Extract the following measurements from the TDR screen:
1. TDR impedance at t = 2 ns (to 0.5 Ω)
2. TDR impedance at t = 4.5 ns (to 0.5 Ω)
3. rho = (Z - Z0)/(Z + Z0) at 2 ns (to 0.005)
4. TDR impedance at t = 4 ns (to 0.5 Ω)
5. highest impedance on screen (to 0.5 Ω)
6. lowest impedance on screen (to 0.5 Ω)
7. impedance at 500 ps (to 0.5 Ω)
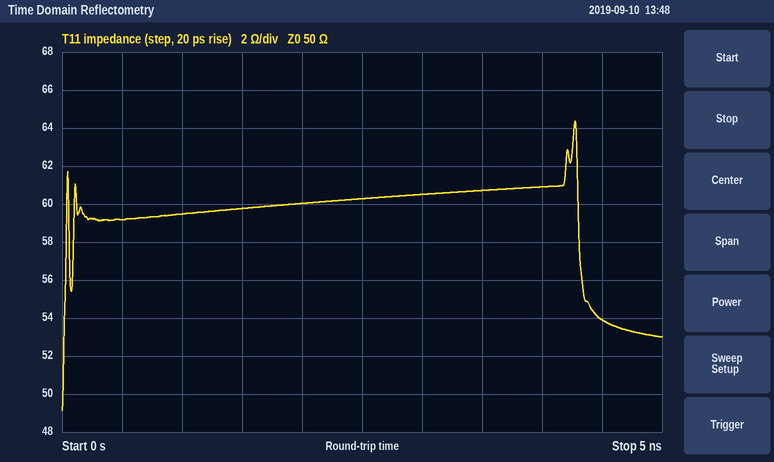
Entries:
60.0 Ω
54.0 Ω
+0.090
61.0 Ω
64.5 Ω
49.0 Ω
59.0 Ω
